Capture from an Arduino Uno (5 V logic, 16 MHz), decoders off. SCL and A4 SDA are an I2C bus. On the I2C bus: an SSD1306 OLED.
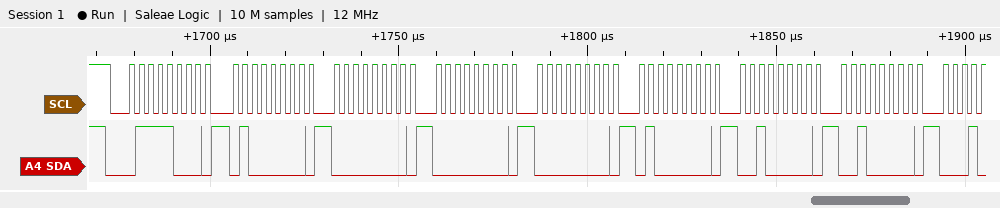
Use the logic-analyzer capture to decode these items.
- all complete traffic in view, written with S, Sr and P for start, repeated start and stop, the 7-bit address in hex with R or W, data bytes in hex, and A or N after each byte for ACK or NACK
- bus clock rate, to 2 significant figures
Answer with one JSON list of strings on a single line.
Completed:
["S 3CW A 40 A 00 A 00 A 00 A 40 A 20 A 20 A", "400 kHz"]
